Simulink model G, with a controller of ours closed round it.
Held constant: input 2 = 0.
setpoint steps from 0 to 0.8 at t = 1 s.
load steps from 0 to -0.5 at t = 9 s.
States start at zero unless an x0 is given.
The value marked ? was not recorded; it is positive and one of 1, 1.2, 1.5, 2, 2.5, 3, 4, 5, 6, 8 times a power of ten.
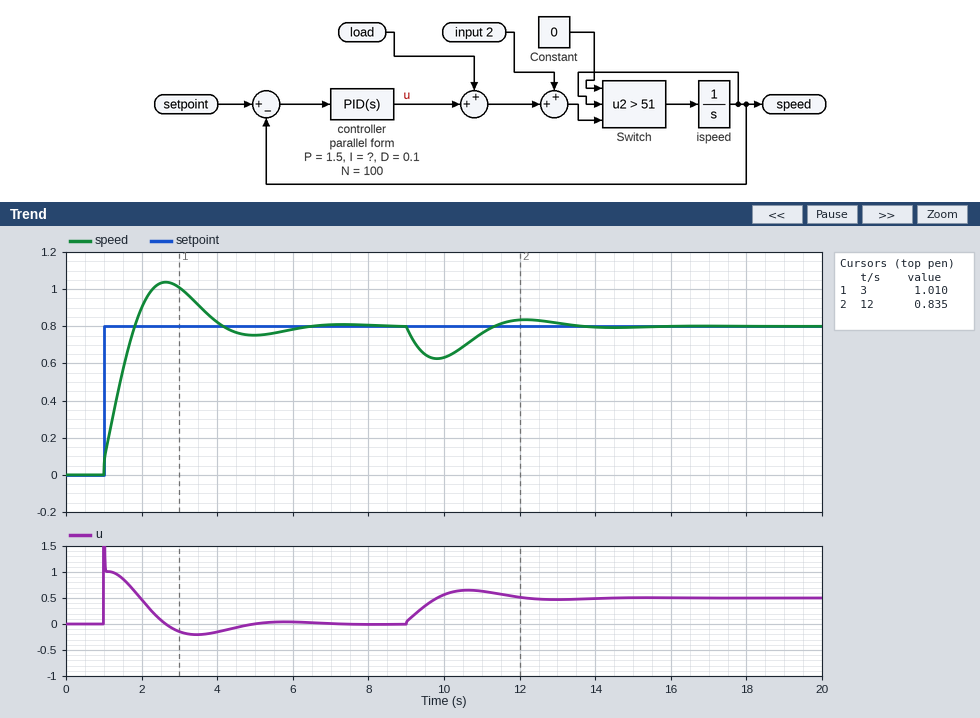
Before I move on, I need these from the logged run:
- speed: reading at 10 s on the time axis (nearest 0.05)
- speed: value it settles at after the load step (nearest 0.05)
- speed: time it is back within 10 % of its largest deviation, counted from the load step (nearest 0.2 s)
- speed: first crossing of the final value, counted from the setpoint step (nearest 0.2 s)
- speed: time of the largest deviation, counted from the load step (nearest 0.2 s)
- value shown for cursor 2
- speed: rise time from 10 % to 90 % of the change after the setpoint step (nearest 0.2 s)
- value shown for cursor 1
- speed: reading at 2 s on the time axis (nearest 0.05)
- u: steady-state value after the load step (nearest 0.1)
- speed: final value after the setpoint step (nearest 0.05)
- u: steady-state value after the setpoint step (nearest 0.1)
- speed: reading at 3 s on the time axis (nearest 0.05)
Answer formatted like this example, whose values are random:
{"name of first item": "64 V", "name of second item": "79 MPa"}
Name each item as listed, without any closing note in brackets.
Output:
{"speed: reading at 10 s on the time axis": "0.65", "speed: value it settles at after the load step": "0.80", "speed: time it is back within 10 % of its largest deviation, counted from the load step": "4.0 s", "speed: first crossing of the final value, counted from the setpoint step": "0.8 s", "speed: time of the largest deviation, counted from the load step": "0.8 s", "value shown for cursor 2": "0.835", "speed: rise time from 10 % to 90 % of the change after the setpoint step": "0.6 s", "value shown for cursor 1": "1.010", "speed: reading at 2 s on the time axis": "0.90", "u: steady-state value after the load step": "0.5", "speed: final value after the setpoint step": "0.80", "u: steady-state value after the setpoint step": "0.0", "speed: reading at 3 s on the time axis": "1.00"}
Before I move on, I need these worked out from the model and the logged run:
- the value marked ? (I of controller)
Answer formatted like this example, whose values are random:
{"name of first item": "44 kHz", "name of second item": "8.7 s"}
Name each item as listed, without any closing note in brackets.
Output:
{"the value marked ?": "2.5"}
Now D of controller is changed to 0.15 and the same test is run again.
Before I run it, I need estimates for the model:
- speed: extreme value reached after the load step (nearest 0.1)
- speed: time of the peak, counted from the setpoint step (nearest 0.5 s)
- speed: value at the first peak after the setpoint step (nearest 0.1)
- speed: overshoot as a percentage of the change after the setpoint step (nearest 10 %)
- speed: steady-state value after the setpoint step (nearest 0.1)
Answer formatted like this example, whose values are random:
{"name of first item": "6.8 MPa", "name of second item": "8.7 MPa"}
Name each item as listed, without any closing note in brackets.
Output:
{"speed: extreme value reached after the load step": "0.6", "speed: time of the peak, counted from the setpoint step": "1.5 s", "speed: value at the first peak after the setpoint step": "1.0", "speed: overshoot as a percentage of the change after the setpoint step": "30 %", "speed: steady-state value after the setpoint step": "0.8"}
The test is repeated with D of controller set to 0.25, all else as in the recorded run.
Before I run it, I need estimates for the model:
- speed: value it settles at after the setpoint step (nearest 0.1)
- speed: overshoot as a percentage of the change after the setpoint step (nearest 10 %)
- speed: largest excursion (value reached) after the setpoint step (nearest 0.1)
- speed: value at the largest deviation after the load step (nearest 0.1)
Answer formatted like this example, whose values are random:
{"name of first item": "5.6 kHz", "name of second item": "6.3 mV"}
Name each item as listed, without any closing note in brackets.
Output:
{"speed: value it settles at after the setpoint step": "0.8", "speed: overshoot as a percentage of the change after the setpoint step": "30 %", "speed: largest excursion (value reached) after the setpoint step": "1.0", "speed: value at the largest deviation after the load step": "0.6"}
